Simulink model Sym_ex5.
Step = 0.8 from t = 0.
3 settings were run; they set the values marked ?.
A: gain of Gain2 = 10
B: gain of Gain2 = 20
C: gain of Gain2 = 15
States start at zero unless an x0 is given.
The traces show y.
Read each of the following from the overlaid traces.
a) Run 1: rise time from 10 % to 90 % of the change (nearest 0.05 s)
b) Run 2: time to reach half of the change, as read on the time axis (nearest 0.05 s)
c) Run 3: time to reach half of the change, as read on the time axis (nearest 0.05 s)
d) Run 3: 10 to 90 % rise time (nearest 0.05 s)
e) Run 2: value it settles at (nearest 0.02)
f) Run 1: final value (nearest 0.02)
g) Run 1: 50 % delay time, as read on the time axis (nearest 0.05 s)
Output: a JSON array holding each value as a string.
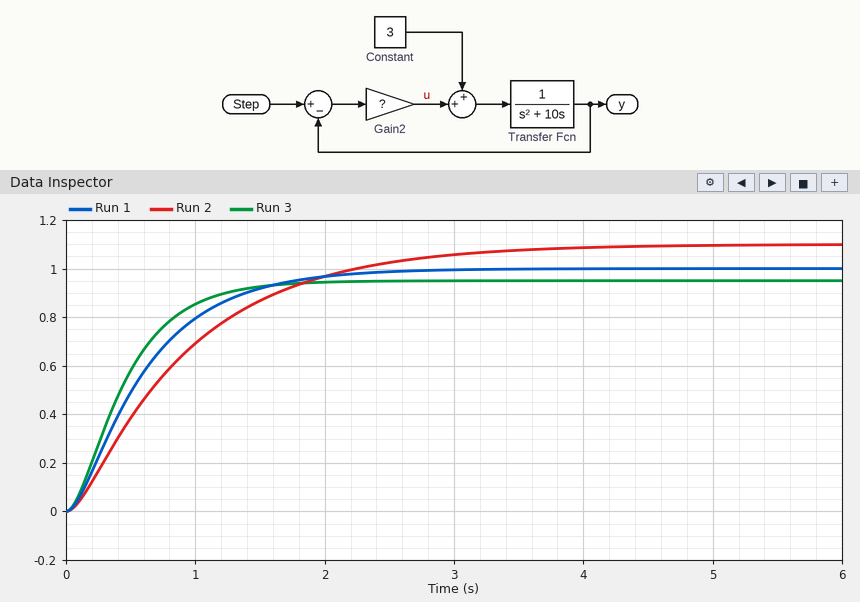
["1.25 s", "0.75 s", "0.40 s", "0.90 s", "1.10", "1.00", "0.50 s"]
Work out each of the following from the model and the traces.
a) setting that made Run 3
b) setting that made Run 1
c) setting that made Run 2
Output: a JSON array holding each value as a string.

["B", "C", "A"]
